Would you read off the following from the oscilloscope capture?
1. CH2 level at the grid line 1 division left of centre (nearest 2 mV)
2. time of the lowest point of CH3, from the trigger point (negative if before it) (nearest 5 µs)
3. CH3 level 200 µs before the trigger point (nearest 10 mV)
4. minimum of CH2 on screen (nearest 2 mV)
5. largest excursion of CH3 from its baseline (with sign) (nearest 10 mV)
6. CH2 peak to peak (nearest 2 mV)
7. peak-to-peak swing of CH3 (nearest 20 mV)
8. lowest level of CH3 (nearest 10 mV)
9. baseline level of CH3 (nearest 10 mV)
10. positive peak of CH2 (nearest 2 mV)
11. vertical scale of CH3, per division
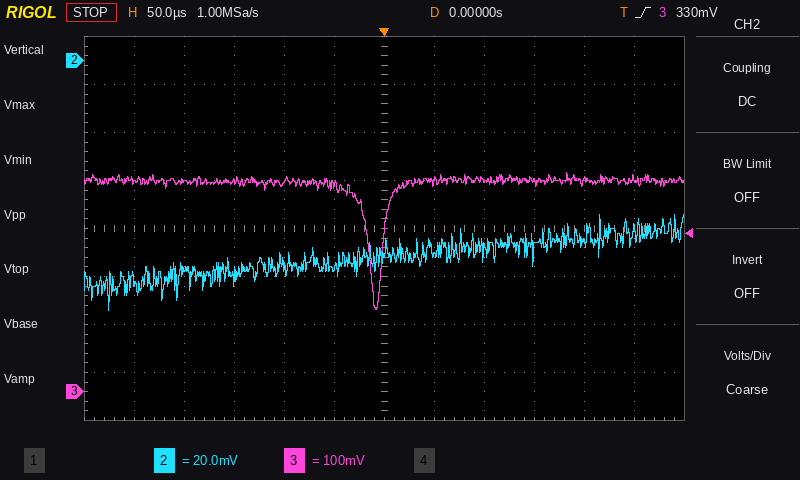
-86 mV
-10 µs
440 mV
-104 mV
-270 mV
40 mV
280 mV
170 mV
440 mV
-64 mV
100 mV
